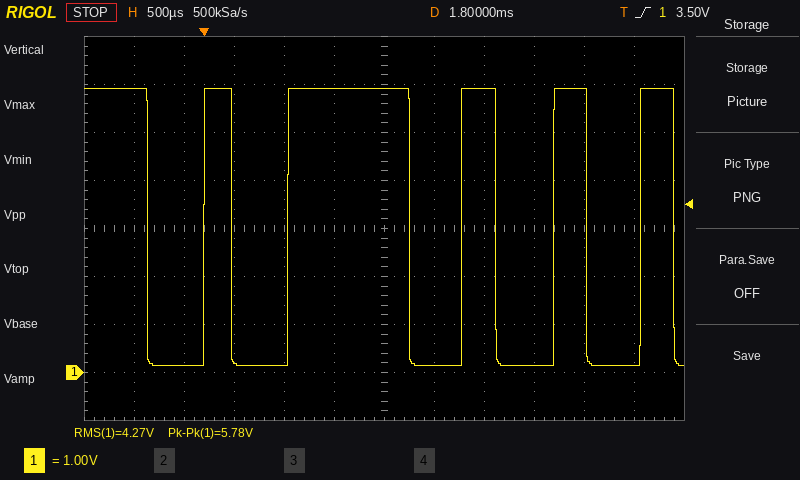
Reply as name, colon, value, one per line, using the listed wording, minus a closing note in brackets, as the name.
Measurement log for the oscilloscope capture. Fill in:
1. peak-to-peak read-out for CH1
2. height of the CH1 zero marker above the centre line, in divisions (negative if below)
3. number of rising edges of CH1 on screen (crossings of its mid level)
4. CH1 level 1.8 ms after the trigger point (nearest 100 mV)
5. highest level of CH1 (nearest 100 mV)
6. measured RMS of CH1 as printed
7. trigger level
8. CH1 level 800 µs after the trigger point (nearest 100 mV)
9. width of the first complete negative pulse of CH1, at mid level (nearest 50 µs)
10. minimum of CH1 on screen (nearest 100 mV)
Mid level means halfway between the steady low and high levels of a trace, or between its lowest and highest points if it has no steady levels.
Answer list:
peak-to-peak read-out for CH1: 5.78 V
height of the CH1 zero marker above the centre line, in divisions: -3.0 div
number of rising edges of CH1 on screen: 5
CH1 level 1.8 ms after the trigger point: 5.9 V
highest level of CH1: 5.9 V
measured RMS of CH1 as printed: 4.27 V
trigger level: 3.50 V
CH1 level 800 µs after the trigger point: 100 mV
width of the first complete negative pulse of CH1, at mid level: 550 µs
minimum of CH1 on screen: 100 mV
